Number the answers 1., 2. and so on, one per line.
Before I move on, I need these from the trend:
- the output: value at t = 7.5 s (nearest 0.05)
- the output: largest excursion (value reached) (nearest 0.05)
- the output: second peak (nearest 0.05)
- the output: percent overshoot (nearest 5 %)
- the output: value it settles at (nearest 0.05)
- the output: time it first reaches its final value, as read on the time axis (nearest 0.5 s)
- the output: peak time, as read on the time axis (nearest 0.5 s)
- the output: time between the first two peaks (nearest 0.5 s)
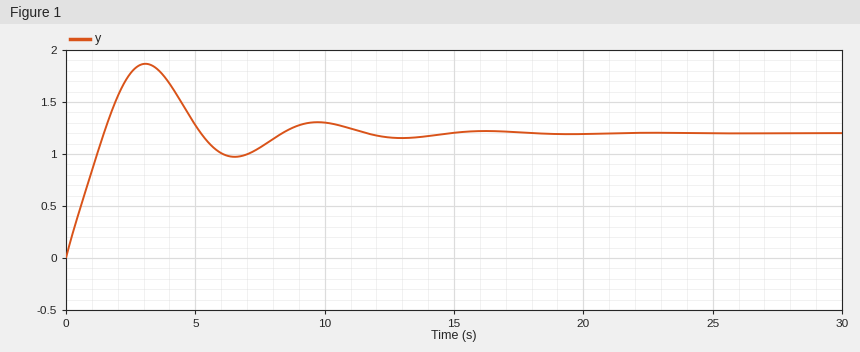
1. 1.05
2. 1.85
3. 1.30
4. 55 %
5. 1.20
6. 1.5 s
7. 3.0 s
8. 6.5 s
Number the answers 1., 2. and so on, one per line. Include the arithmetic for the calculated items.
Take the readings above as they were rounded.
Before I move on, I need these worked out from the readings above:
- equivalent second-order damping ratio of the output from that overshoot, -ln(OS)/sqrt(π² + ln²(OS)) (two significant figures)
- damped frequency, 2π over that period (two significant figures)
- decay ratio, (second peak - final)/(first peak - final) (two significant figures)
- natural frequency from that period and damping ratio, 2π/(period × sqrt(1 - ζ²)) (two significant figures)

1. ln(0.55) = -0.598; 0.598 / sqrt(9.870 + 0.357) = 0.19
2. 2π / 6.5 = 0.97 rad/s
3. (1.3 - 1.2) / (1.85 - 1.2) = 0.15
4. 2π / (6.5 × sqrt(1 - 0.19²)) = 0.98 rad/s
